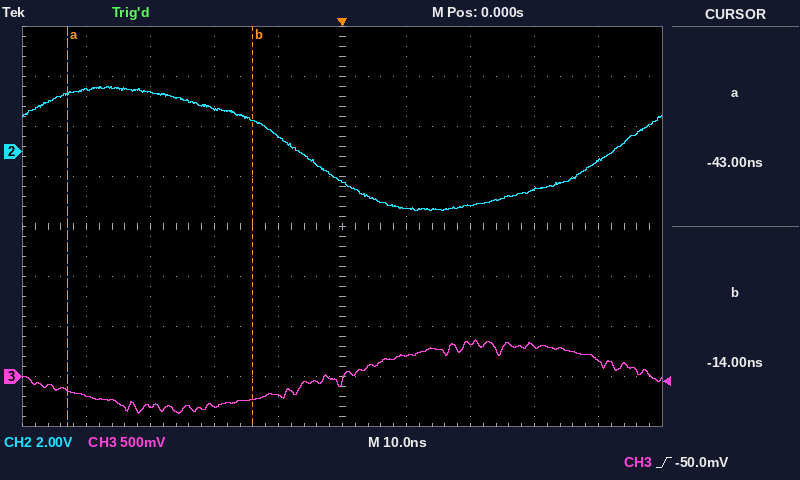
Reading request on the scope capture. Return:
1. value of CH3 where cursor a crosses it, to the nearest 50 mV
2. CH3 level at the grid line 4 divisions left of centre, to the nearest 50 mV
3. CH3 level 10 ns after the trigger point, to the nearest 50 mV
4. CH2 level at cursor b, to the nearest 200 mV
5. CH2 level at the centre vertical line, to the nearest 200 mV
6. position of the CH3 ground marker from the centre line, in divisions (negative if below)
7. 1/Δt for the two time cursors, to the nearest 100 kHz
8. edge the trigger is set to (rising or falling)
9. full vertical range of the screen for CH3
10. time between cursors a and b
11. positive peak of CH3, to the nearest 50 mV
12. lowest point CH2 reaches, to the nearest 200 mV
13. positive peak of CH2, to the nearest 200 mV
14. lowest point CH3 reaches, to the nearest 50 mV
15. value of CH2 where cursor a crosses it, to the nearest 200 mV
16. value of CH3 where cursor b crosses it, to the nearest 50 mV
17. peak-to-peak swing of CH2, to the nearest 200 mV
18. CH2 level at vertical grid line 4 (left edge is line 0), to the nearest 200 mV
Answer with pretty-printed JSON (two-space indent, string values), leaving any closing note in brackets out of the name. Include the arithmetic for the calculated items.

{
  "value of CH3 where cursor a crosses it, to the nearest 50 mV": "-150 mV",
  "CH3 level at the grid line 4 divisions left of centre, to the nearest 50 mV": "-200 mV",
  "CH3 level 10 ns after the trigger point, to the nearest 50 mV": "200 mV",
  "CH2 level at cursor b, to the nearest 200 mV": "1.2 V",
  "CH2 level at the centre vertical line, to the nearest 200 mV": "-1.2 V",
  "position of the CH3 ground marker from the centre line, in divisions": "-3.0 div",
  "1/Δt for the two time cursors, to the nearest 100 kHz": "1 / 29 ns ≈ 34.5 MHz",
  "edge the trigger is set to": "rising",
  "full vertical range of the screen for CH3": "4 V",
  "time between cursors a and b": "-14 ns − (-43 ns) = 29 ns",
  "positive peak of CH3, to the nearest 50 mV": "350 mV",
  "lowest point CH2 reaches, to the nearest 200 mV": "-2.4 V",
  "positive peak of CH2, to the nearest 200 mV": "2.6 V",
  "lowest point CH3 reaches, to the nearest 50 mV": "-350 mV",
  "value of CH2 where cursor a crosses it, to the nearest 200 mV": "2.4 V",
  "value of CH3 where cursor b crosses it, to the nearest 50 mV": "-250 mV",
  "peak-to-peak swing of CH2, to the nearest 200 mV": "2.6 V − (-2.4 V) = 5.0 V",
  "CH2 level at vertical grid line 4 (left edge is line 0), to the nearest 200 mV": "600 mV"
}
